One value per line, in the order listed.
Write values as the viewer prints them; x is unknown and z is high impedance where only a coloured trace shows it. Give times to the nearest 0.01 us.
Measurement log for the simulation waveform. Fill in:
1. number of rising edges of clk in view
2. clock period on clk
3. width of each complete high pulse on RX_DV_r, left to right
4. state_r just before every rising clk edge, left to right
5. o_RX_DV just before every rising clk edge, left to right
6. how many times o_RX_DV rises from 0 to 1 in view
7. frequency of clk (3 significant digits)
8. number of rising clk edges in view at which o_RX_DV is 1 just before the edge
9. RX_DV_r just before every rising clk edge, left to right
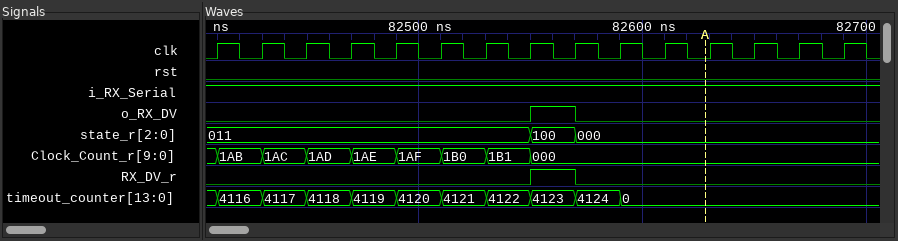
15
0.02 us
0.02 us
011, 011, 011, 011, 011, 011, 011, 011, 100, 000, 000, 000, 000, 000, 000
0 0 0 0 0 0 0 0 1 0 0 0 0 0 0
1
50.0 MHz
1
0 0 0 0 0 0 0 0 1 0 0 0 0 0 0
